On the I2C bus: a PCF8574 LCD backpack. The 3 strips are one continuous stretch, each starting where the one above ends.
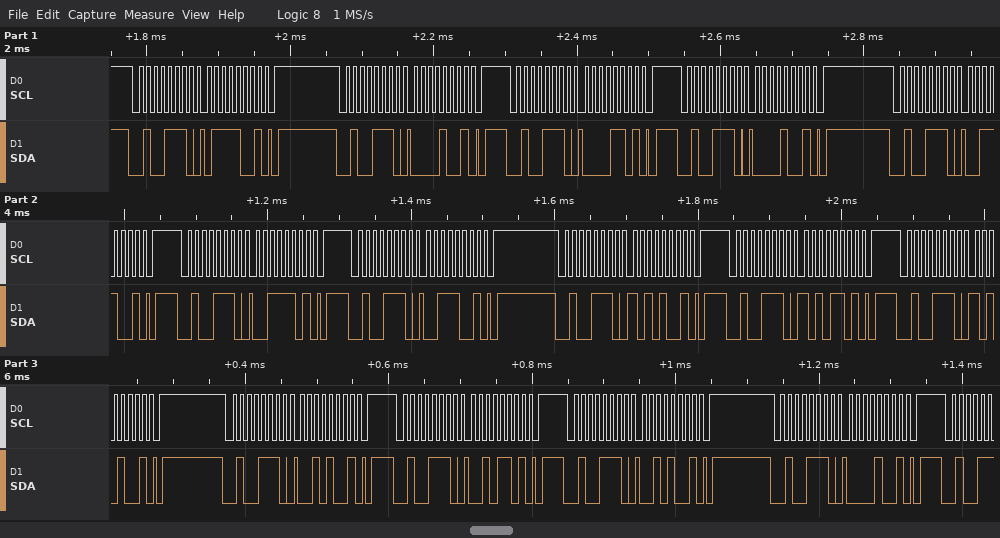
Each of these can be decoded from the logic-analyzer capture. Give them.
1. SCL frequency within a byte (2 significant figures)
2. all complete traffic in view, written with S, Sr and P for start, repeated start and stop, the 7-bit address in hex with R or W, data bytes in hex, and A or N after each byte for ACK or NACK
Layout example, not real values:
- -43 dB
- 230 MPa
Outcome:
- 100 kHz
- S 27W A 79 A P S 27W A 09 A P S 27W A 0D A P S 27W A 09 A P S 27W A 39 A P S 27W A 3D A P S 27W A 39 A P S 27W A A9 A P S 27W A AD A P S 27W A A9 A P S 27W A 29 A P S 27W A 2D A P S 27W A 29 A P S 27W A 09 A P
